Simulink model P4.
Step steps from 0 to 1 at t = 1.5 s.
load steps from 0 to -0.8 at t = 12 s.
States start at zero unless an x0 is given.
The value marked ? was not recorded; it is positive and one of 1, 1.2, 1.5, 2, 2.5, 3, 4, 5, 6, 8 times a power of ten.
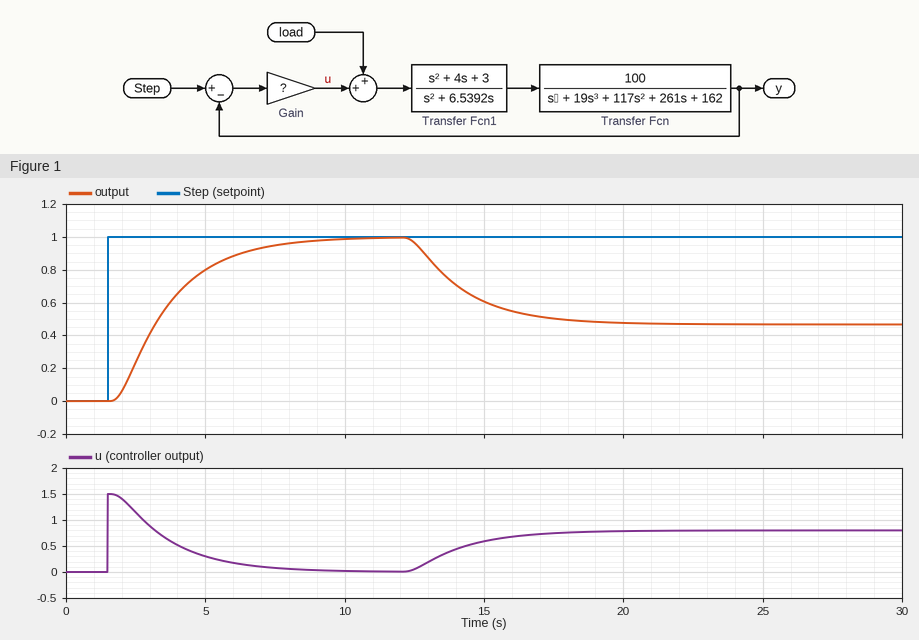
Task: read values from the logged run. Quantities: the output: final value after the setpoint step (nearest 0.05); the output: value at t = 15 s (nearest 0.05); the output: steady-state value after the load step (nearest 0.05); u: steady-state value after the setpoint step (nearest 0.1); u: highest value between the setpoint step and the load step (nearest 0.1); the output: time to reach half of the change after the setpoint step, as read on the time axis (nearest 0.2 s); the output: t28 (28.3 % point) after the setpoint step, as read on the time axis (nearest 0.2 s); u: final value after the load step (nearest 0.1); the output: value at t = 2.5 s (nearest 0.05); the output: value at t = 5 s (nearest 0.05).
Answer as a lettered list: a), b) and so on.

a) 1.00
b) 0.60
c) 0.45
d) 0.0
e) 1.5
f) 3.4 s
g) 2.6 s
h) 0.8
i) 0.25
j) 0.80
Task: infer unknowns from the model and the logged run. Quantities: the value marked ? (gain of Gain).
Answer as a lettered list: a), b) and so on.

a) 1.5
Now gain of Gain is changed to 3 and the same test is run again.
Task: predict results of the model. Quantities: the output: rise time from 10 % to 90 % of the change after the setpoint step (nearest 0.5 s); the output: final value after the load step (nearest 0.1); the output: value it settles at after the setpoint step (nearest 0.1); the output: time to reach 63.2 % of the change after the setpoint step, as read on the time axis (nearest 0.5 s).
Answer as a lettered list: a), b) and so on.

a) 1.5 s
b) 0.7
c) 1.0
d) 3.0 s
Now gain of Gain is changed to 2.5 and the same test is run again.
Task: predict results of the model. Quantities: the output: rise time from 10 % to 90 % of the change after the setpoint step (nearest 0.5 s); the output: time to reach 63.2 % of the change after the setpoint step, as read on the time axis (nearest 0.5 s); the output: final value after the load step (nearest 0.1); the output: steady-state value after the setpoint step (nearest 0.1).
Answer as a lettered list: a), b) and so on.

a) 2.0 s
b) 3.0 s
c) 0.7
d) 1.0
